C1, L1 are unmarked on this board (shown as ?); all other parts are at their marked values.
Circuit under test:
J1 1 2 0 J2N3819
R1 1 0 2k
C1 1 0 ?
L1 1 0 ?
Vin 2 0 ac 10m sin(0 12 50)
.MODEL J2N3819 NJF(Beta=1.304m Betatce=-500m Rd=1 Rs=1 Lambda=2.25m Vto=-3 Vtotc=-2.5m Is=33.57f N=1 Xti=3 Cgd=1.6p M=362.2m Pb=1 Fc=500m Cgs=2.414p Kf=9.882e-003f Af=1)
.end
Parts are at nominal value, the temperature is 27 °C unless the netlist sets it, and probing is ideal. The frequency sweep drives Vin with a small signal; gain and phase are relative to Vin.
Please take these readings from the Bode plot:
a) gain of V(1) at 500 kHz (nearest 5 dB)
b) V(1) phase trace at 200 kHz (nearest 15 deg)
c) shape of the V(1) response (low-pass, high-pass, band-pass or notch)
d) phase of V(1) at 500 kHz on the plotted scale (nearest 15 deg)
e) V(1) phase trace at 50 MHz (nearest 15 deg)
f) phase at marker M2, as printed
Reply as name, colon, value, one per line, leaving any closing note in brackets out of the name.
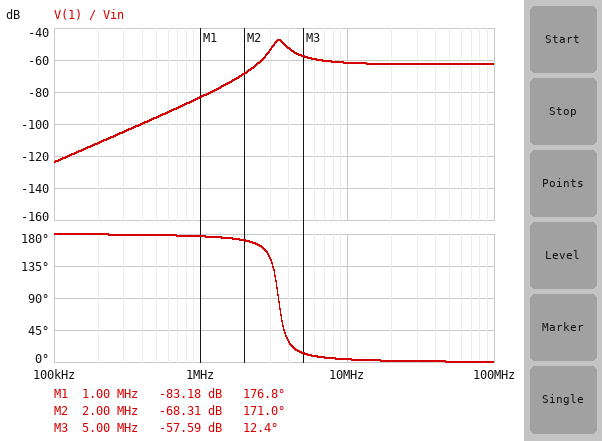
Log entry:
gain of V(1) at 500 kHz: -95 dB
V(1) phase trace at 200 kHz: 180 deg
shape of the V(1) response: high-pass
phase of V(1) at 500 kHz on the plotted scale: 180 deg
V(1) phase trace at 50 MHz: 0 deg
phase at marker M2, as printed: 171.0 deg
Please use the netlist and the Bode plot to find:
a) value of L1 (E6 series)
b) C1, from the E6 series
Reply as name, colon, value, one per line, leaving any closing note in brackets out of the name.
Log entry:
value of L1: 1 µH
C1, from the E6 series: 2.2 nF
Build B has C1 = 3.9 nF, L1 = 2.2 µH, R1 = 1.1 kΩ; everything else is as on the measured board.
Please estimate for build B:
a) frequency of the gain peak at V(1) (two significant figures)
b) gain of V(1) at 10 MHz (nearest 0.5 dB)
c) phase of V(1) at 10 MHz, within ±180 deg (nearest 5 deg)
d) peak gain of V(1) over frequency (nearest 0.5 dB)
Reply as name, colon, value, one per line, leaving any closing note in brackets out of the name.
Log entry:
frequency of the gain peak at V(1): 1.7 MHz
gain of V(1) at 10 MHz: -67.5 dB
phase of V(1) at 10 MHz, within ±180 deg: 0 deg
peak gain of V(1) over frequency: -54.0 dB
